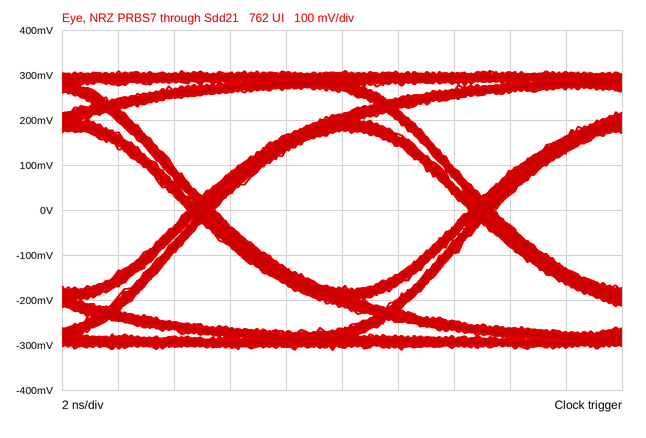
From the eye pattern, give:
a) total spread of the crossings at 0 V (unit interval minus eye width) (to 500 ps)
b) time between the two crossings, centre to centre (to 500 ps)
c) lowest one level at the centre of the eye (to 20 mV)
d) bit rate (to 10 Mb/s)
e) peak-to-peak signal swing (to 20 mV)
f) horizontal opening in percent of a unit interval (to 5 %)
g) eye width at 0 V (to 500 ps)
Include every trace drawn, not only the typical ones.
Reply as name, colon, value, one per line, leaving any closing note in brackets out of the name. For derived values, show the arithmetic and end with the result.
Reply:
total spread of the crossings at 0 V (unit interval minus eye width): 1.0 ns
time between the two crossings, centre to centre: 10.0 ns
lowest one level at the centre of the eye: 180 mV
bit rate: 100 Mb/s
peak-to-peak signal swing: 620 mV
horizontal opening in percent of a unit interval: 9.0 ns / 10.0 ns ≈ 90 %
eye width at 0 V: 9.0 ns
